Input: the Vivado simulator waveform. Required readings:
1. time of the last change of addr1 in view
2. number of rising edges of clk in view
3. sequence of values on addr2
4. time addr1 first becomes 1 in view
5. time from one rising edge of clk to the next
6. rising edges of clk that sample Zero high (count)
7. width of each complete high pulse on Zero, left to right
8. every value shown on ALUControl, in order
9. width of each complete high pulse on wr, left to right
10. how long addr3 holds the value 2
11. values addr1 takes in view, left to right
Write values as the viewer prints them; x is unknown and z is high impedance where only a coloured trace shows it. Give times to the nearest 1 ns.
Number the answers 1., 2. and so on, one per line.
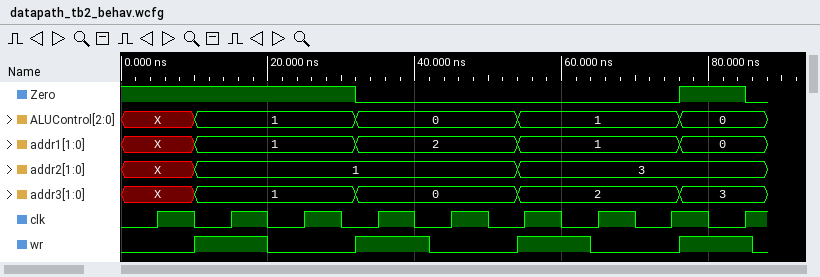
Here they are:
1. 76 ns
2. 9
3. X, 1, 3
4. 10 ns
5. 10 ns
6. 4
7. 9 ns
8. X, 1, 0, 1, 0
9. 10 ns, 10 ns, 10 ns, 10 ns
10. 22 ns
11. X, 1, 2, 1, 0
